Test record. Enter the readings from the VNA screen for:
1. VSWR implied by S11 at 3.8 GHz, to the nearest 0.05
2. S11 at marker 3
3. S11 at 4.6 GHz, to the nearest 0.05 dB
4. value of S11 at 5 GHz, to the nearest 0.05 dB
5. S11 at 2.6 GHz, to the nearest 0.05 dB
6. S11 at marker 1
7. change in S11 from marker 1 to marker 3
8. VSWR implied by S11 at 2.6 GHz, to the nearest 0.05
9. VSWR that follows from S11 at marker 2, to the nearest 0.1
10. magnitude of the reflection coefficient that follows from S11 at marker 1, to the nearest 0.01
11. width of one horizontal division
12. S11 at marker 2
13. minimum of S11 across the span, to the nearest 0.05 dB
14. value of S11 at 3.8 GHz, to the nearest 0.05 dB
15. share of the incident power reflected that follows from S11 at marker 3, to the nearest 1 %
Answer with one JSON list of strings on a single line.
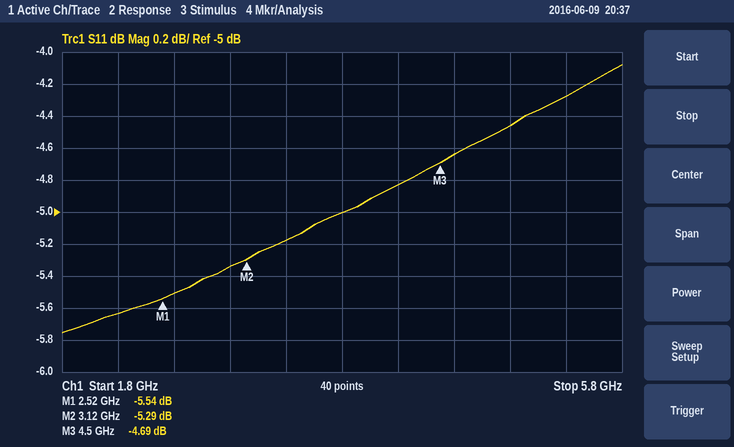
["3.55", "-4.69 dB", "-4.65 dB", "-4.45 dB", "-5.50 dB", "-5.54 dB", "0.85 dB", "3.25", "3.4", "0.53", "400 MHz", "-5.29 dB", "-5.75 dB", "-5.00 dB", "34 %"]
